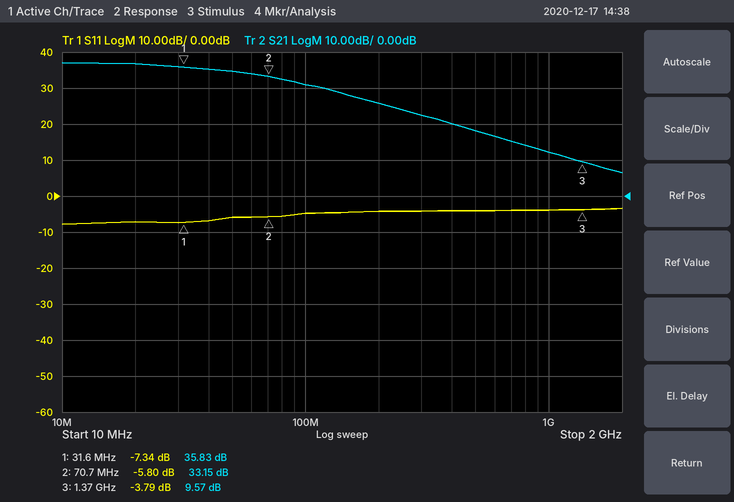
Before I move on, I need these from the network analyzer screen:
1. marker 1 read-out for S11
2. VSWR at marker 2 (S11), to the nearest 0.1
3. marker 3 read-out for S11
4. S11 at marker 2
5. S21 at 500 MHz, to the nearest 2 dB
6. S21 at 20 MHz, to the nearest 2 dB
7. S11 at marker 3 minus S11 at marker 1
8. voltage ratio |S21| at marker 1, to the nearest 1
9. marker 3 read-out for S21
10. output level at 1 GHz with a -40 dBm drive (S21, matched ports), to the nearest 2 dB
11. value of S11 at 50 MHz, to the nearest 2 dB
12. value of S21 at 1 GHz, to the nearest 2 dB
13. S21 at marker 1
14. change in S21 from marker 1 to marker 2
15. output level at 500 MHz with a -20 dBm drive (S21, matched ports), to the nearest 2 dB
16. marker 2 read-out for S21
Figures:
-7.34 dB
3.1
-3.79 dB
-5.80 dB
18 dB
36 dB
3.55 dB
62
9.57 dB
-28 dBm
-6 dB
12 dB
35.83 dB
-2.68 dB
-2 dBm
33.15 dB
